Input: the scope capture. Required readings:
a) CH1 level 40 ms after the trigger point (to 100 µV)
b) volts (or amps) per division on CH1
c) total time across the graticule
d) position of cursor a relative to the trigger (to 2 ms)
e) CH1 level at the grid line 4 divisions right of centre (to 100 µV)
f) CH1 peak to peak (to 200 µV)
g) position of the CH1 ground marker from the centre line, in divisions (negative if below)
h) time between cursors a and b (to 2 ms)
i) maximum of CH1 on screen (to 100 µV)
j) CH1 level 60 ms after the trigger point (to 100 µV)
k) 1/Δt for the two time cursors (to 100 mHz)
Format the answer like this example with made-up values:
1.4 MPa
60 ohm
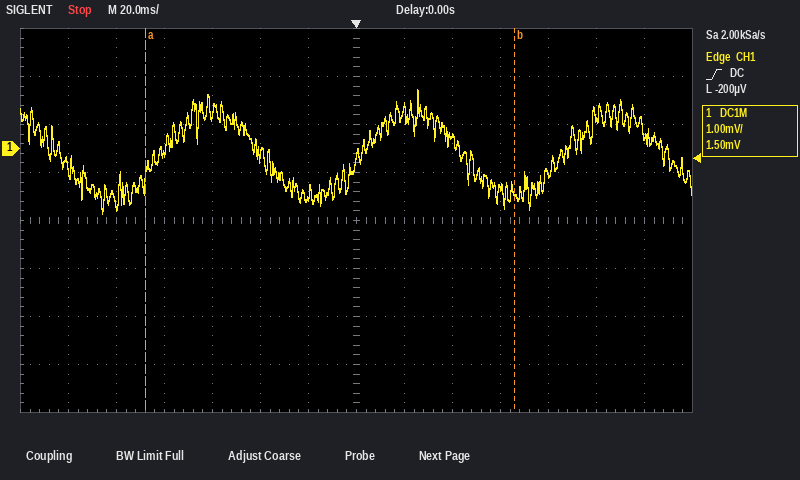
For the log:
300 µV
1 mV
280 ms
-88 ms
-500 µV
2.6 mV
+1.5 div
154 ms
1.2 mV
-800 µV
6.5 Hz
